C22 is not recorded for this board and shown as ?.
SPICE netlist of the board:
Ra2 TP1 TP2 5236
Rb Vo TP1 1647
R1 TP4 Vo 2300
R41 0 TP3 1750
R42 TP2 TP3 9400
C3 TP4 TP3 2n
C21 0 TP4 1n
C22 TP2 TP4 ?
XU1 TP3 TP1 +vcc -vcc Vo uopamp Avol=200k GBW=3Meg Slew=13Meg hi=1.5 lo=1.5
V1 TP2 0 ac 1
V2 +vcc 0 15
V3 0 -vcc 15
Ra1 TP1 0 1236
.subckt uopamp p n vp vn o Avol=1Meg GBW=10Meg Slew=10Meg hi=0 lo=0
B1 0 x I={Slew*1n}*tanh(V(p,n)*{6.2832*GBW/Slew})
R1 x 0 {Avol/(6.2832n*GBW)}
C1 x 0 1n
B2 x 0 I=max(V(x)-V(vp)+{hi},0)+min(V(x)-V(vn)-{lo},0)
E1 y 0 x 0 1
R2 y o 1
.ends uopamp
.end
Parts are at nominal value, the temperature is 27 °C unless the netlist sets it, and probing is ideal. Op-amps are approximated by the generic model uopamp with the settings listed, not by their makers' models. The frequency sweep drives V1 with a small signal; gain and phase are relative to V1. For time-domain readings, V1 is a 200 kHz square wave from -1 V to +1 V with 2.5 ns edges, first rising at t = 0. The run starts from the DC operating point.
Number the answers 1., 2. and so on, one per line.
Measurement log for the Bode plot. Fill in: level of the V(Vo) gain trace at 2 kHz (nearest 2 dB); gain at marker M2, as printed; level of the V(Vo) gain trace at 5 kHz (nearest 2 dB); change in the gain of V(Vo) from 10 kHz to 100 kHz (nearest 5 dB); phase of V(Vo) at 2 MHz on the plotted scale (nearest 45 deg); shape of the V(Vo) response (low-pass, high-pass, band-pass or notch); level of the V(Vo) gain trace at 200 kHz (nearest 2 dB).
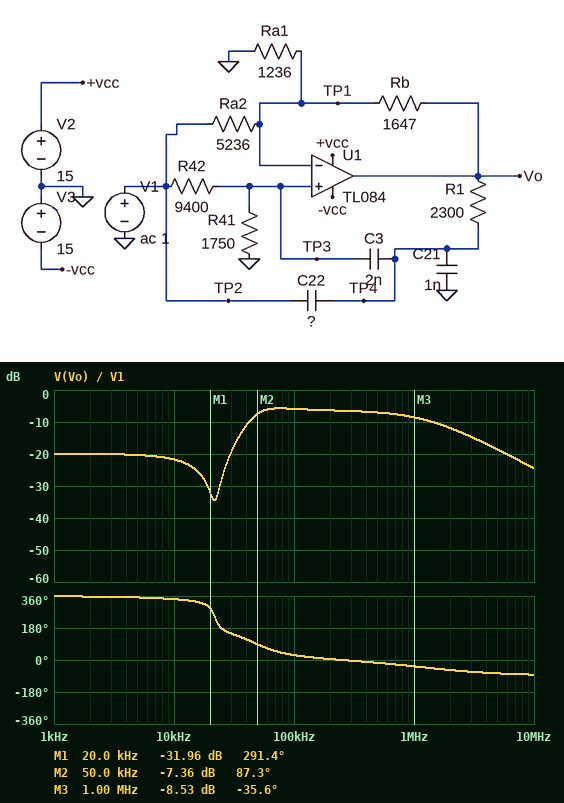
1. -20 dB
2. -7.36 dB
3. -20 dB
4. 15 dB
5. -45 deg
6. band-pass
7. -6 dB
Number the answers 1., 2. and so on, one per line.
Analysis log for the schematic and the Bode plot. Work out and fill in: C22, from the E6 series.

1. 470 pF
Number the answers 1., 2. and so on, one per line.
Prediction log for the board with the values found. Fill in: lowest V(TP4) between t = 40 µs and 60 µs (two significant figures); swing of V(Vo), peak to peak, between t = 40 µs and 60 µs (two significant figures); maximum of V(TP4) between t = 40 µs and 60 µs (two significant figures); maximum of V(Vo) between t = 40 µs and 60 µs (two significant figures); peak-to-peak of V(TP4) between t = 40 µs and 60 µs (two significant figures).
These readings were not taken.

1. -350 mV
2. 1.2 V
3. 350 mV
4. 590 mV
5. 710 mV
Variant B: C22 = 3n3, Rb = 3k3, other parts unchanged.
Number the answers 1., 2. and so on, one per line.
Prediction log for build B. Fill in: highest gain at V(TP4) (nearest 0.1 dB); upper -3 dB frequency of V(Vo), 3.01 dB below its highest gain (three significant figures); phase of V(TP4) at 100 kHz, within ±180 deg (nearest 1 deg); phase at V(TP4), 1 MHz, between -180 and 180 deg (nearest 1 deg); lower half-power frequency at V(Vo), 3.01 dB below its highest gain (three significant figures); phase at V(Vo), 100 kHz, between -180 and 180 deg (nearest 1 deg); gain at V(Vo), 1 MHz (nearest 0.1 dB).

1. 4.0 dB
2. 344 kHz
3. -9 deg
4. 1 deg
5. 23.8 kHz
6. 8 deg
7. 3.4 dB
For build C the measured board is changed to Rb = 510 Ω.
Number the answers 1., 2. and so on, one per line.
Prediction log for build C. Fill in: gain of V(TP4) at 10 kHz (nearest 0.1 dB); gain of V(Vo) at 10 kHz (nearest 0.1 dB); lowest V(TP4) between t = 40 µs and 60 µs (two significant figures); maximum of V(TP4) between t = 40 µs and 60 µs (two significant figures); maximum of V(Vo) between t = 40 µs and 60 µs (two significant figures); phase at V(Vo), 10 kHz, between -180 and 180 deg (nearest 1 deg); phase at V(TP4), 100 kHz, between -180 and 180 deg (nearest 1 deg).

1. -16.4 dB
2. -17.8 dB
3. -390 mV
4. 390 mV
5. 480 mV
6. -1 deg
7. 13 deg
